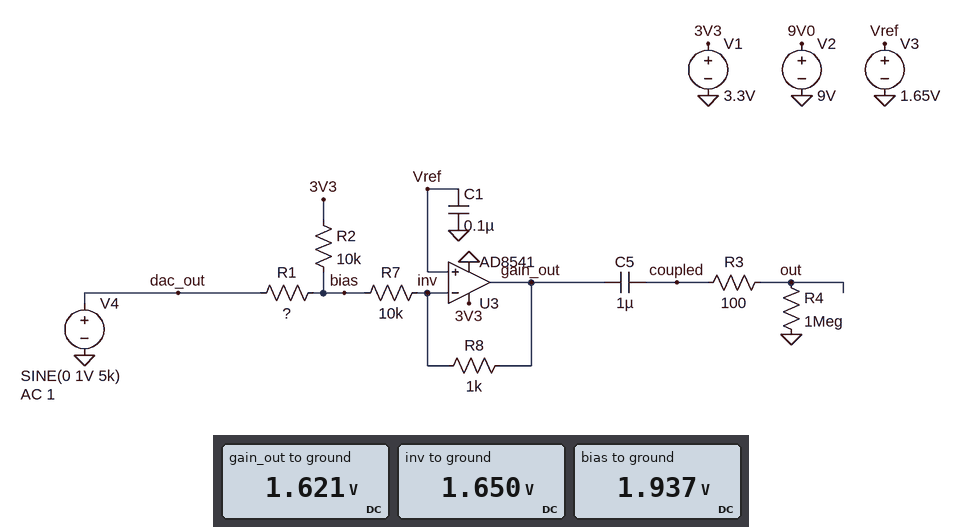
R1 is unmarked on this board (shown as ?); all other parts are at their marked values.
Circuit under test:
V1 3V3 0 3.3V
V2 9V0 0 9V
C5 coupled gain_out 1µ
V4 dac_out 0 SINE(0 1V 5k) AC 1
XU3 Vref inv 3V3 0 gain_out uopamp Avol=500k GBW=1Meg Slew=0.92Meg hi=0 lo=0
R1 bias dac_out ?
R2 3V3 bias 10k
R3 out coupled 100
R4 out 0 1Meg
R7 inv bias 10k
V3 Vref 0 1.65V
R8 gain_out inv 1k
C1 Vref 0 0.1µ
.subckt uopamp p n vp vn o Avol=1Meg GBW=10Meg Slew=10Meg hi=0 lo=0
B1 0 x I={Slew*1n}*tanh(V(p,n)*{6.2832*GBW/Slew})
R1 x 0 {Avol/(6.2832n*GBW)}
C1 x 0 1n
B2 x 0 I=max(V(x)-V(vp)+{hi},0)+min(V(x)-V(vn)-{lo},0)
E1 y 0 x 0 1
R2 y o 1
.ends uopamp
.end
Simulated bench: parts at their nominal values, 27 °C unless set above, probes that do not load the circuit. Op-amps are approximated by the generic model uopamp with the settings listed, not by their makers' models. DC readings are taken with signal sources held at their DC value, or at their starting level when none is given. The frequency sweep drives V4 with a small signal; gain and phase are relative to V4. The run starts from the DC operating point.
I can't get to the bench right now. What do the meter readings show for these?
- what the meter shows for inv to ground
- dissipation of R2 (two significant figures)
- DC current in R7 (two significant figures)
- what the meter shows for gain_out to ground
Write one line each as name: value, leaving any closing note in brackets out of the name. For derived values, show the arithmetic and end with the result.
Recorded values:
what the meter shows for inv to ground: 1.650 V
dissipation of R2: (3.3 V - 1.937 V)^2 / 10 kΩ = 190 µW
DC current in R7: (1.937 V - 1.65 V) / 10 kΩ = 29 µA
what the meter shows for gain_out to ground: 1.621 V
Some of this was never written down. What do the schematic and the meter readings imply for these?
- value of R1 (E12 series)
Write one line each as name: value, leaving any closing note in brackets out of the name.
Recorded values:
value of R1: 18 kΩ
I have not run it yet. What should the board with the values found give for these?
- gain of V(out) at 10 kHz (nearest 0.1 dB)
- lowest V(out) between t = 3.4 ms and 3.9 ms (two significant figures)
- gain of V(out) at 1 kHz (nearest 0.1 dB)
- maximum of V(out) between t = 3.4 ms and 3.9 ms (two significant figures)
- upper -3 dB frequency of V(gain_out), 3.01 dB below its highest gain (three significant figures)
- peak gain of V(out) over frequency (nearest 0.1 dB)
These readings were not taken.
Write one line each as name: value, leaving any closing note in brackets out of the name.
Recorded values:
gain of V(out) at 10 kHz: -33.3 dB
lowest V(out) between t = 3.4 ms and 3.9 ms: -22 mV
gain of V(out) at 1 kHz: -33.3 dB
maximum of V(out) between t = 3.4 ms and 3.9 ms: 22 mV
upper -3 dB frequency of V(gain_out), 3.01 dB below its highest gain: 943 kHz
peak gain of V(out) over frequency: -33.3 dB
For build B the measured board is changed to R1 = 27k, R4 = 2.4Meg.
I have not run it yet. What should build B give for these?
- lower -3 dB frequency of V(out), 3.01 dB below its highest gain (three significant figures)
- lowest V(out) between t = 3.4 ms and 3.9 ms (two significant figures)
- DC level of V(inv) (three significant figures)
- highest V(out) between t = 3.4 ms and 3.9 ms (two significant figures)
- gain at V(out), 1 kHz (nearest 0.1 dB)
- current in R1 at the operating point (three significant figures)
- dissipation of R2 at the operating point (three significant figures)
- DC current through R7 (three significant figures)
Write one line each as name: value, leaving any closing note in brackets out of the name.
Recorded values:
lower -3 dB frequency of V(out), 3.01 dB below its highest gain: 66.3 mHz
lowest V(out) between t = 3.4 ms and 3.9 ms: -16 mV
DC level of V(inv): 1.65 V
highest V(out) between t = 3.4 ms and 3.9 ms: 16 mV
gain at V(out), 1 kHz: -36.1 dB
current in R1 at the operating point: 77.3 µA
dissipation of R2 at the operating point: 147 µW
DC current through R7: 43.8 µA
